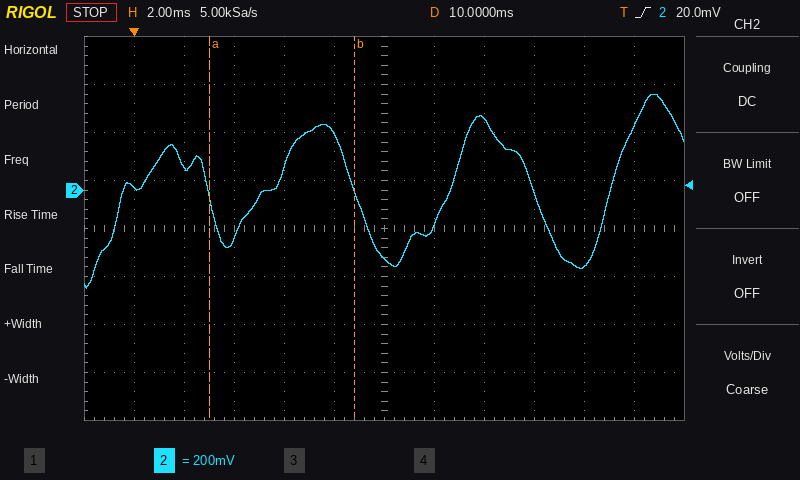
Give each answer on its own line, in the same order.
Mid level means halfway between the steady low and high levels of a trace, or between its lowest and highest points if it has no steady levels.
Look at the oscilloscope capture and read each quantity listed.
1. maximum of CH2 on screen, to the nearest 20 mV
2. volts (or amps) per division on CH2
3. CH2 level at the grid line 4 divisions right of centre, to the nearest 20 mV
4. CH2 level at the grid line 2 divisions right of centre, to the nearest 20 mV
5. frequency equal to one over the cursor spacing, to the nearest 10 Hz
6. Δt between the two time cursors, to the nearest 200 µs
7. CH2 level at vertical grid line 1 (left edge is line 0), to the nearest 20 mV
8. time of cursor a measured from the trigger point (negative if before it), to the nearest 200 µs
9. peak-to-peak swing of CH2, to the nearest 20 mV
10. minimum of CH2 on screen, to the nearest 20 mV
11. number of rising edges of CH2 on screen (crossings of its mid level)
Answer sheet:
400 mV
200 mV
-320 mV
300 mV
170 Hz
5.8 ms
20 mV
+3.0 ms
800 mV
-400 mV
4
